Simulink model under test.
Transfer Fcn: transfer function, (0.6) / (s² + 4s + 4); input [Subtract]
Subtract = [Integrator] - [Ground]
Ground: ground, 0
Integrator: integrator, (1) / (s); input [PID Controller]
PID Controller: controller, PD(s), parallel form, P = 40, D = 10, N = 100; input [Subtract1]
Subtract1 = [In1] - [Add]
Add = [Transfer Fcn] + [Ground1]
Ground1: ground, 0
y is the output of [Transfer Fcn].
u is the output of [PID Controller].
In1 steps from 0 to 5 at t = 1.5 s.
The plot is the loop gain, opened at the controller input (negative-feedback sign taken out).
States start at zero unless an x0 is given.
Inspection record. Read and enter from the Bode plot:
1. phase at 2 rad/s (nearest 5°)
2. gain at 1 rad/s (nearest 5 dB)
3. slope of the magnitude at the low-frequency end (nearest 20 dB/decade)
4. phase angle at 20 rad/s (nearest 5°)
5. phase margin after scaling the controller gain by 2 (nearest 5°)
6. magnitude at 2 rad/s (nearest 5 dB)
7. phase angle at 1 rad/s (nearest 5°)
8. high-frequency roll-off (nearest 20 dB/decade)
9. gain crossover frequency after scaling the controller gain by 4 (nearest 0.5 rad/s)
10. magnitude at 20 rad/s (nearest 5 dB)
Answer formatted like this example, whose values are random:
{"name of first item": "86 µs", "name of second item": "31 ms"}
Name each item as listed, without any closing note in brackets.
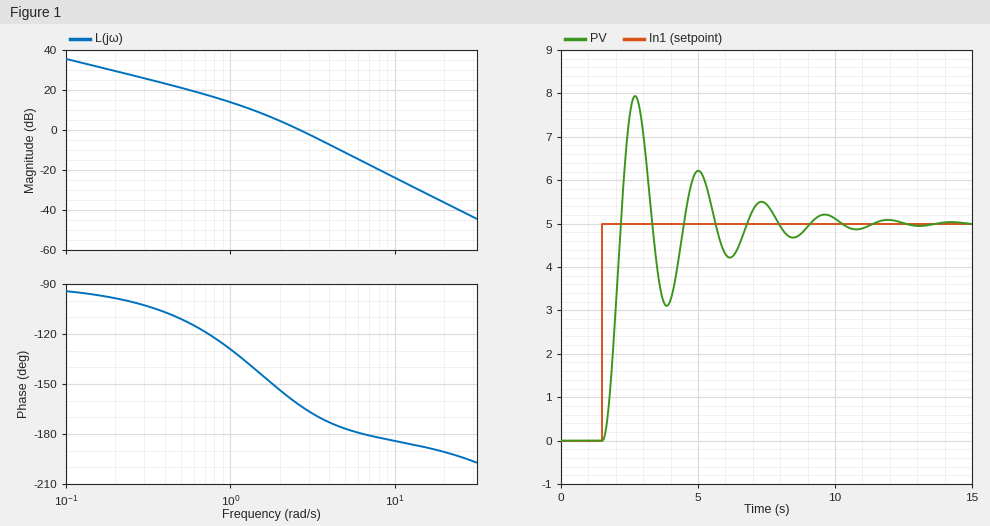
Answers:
{"phase at 2 rad/s": "-155°", "gain at 1 rad/s": "15 dB", "slope of the magnitude at the low-frequency end": "-20 dB/decade", "phase angle at 20 rad/s": "-190°", "phase margin after scaling the controller gain by 2": "10°", "magnitude at 2 rad/s": "5 dB", "phase angle at 1 rad/s": "-130°", "high-frequency roll-off": "-40 dB/decade", "gain crossover frequency after scaling the controller gain by 4": "5.0 rad/s", "magnitude at 20 rad/s": "-35 dB"}
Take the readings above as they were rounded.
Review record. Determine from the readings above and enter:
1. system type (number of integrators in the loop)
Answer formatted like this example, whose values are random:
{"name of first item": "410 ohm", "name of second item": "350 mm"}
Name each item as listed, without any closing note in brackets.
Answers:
{"system type": "1"}
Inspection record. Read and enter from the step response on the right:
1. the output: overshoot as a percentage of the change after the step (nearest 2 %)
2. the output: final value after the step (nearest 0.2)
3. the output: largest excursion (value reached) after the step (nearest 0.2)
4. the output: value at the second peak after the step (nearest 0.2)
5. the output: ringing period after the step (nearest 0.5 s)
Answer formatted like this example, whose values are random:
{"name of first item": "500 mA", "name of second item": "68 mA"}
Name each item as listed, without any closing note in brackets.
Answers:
{"the output: overshoot as a percentage of the change after the step": "58 %", "the output: final value after the step": "5.0", "the output: largest excursion (value reached) after the step": "8.0", "the output: value at the second peak after the step": "6.2", "the output: ringing period after the step": "2.5 s"}
